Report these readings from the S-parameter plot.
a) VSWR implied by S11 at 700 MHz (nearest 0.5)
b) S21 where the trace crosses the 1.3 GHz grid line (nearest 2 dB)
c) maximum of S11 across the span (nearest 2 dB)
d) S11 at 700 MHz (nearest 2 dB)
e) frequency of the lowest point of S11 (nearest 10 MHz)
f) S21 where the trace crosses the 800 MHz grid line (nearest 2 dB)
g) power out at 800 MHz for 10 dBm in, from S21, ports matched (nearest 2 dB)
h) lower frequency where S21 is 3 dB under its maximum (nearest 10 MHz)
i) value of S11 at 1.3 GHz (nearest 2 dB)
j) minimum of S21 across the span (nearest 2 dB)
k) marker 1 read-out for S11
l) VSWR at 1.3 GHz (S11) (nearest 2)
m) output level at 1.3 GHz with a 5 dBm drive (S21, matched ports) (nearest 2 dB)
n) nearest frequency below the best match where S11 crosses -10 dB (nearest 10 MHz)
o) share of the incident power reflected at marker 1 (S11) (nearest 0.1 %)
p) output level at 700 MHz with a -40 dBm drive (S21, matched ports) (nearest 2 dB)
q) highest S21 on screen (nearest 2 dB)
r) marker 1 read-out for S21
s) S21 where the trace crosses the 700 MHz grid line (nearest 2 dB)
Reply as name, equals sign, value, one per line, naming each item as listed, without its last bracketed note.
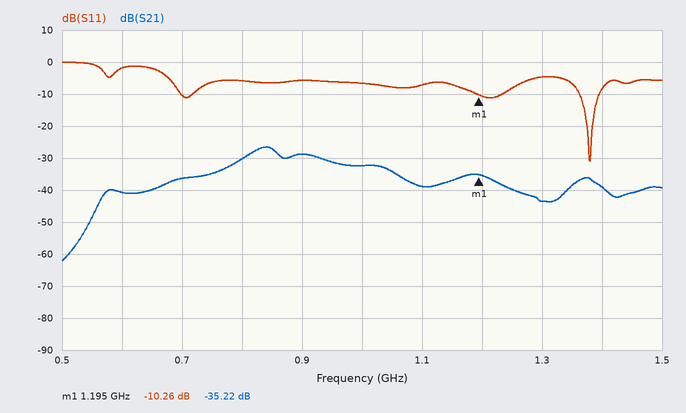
VSWR implied by S11 at 700 MHz = 2.0
S21 where the trace crosses the 1.3 GHz grid line = -44 dB
maximum of S11 across the span = 0 dB
S11 at 700 MHz = -10 dB
frequency of the lowest point of S11 = 1.38 GHz
S21 where the trace crosses the 800 MHz grid line = -30 dB
power out at 800 MHz for 10 dBm in, from S21, ports matched = -20 dBm
lower frequency where S21 is 3 dB under its maximum = 810 MHz
value of S11 at 1.3 GHz = -4 dB
minimum of S21 across the span = -62 dB
marker 1 read-out for S11 = -10.26 dB
VSWR at 1.3 GHz (S11) = 4
output level at 1.3 GHz with a 5 dBm drive (S21, matched ports) = -38 dBm
nearest frequency below the best match where S11 crosses -10 dB = 1.36 GHz
share of the incident power reflected at marker 1 (S11) = 9.4 %
output level at 700 MHz with a -40 dBm drive (S21, matched ports) = -76 dBm
highest S21 on screen = -26 dB
marker 1 read-out for S21 = -35.22 dB
S21 where the trace crosses the 700 MHz grid line = -36 dB
